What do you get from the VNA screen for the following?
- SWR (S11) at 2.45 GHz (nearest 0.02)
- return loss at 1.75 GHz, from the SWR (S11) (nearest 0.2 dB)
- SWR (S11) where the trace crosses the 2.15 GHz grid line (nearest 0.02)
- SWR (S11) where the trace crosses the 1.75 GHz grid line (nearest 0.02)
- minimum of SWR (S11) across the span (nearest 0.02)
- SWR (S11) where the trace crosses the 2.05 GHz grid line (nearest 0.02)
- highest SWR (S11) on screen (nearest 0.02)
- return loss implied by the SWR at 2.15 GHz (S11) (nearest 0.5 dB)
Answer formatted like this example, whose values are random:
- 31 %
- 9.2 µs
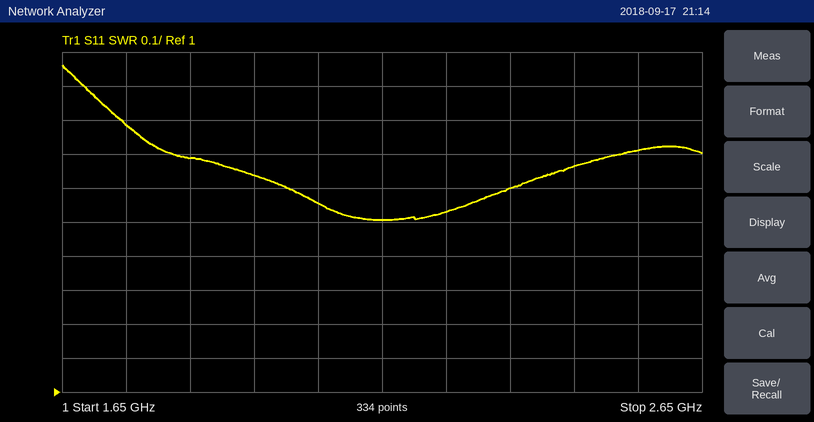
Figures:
- 1.66
- 11.0 dB
- 1.50
- 1.78
- 1.50
- 1.56
- 1.96
- 14.0 dB
